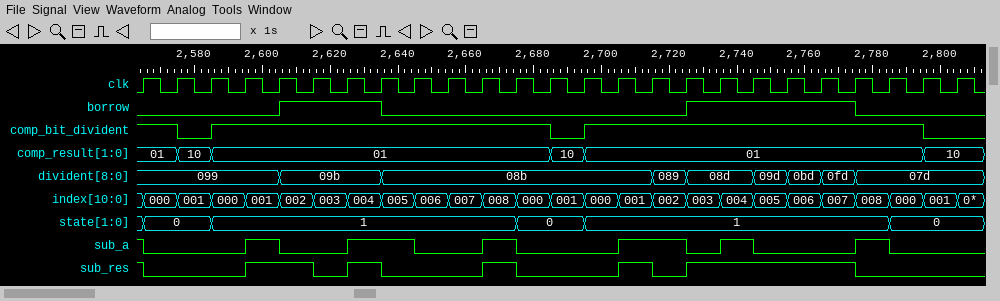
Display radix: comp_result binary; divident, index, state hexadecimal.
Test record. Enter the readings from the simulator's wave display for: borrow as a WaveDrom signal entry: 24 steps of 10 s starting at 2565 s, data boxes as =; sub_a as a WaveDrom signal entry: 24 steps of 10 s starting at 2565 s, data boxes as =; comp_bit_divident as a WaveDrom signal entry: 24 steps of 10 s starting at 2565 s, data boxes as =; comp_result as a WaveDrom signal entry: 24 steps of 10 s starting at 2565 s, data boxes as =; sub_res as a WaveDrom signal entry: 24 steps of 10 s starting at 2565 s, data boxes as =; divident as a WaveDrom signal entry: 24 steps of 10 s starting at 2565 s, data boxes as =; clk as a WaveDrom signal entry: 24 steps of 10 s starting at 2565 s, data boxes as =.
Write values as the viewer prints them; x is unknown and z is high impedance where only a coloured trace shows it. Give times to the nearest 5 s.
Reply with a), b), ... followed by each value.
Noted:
a) {name: 'borrow', wave: '0...1..0........1....0..'}
b) {name: 'sub_a', wave: '0..10.1.0.10..1.010..10.'}
c) {name: 'comp_bit_divident', wave: '101.........01.........0'}
d) {name: 'comp_result', wave: '===.........==.........=', data: '01 10 01 10 01 10'}
e) {name: 'sub_res', wave: '0..1.010..10..101....0..'}
f) {name: 'divident', wave: '=...=..=.......==.====..', data: '099 09b 08b 089 08d 09d 0bd 0fd 07d'}
g) {name: 'clk', wave: 'p.......................'}
